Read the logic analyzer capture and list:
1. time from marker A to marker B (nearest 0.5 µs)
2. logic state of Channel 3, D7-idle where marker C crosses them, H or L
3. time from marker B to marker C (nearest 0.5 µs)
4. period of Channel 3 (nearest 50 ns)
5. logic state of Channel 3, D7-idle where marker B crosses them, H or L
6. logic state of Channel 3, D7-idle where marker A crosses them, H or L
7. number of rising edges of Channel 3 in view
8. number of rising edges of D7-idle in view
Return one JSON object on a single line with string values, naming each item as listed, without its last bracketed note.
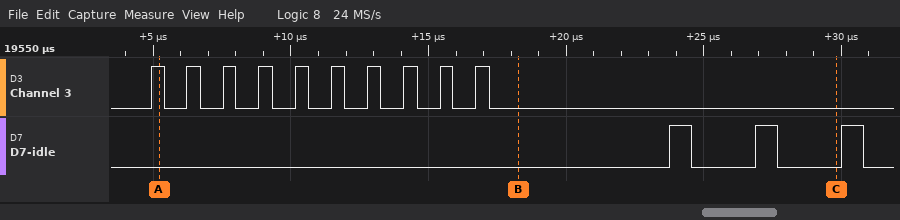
{"time from marker A to marker B": "13 µs", "logic state of Channel 3, D7-idle where marker C crosses them, H or L": "Channel 3=L, D7-idle=L", "time from marker B to marker C": "11.5 µs", "period of Channel 3": "1300 ns", "logic state of Channel 3, D7-idle where marker B crosses them, H or L": "Channel 3=L, D7-idle=L", "logic state of Channel 3, D7-idle where marker A crosses them, H or L": "Channel 3=H, D7-idle=L", "number of rising edges of Channel 3 in view": "10", "number of rising edges of D7-idle in view": "3"}
